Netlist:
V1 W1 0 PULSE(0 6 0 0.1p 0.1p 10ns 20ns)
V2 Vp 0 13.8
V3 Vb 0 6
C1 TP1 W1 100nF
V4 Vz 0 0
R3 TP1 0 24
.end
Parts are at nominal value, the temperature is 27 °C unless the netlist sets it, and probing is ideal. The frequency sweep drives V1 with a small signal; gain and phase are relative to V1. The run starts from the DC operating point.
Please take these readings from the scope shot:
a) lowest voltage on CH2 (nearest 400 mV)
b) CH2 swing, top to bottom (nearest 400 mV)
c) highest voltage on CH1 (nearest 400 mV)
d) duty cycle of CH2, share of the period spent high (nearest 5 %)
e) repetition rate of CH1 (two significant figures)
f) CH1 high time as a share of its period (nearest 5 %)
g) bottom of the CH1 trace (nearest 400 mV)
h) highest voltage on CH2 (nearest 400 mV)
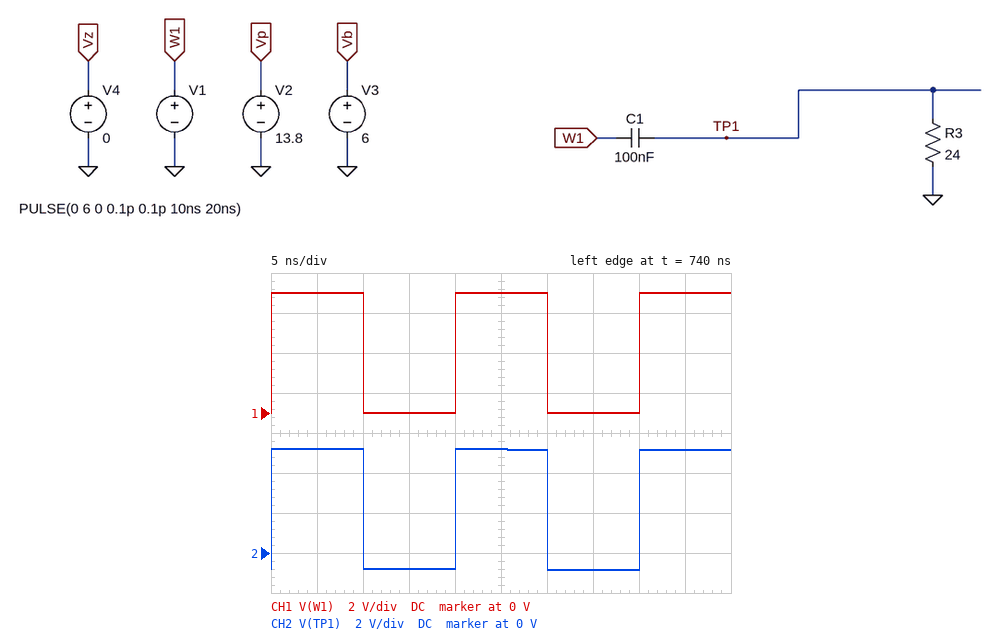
-800 mV
6.0 V
6.0 V
50 %
50 MHz
50 %
0 V
5.2 V
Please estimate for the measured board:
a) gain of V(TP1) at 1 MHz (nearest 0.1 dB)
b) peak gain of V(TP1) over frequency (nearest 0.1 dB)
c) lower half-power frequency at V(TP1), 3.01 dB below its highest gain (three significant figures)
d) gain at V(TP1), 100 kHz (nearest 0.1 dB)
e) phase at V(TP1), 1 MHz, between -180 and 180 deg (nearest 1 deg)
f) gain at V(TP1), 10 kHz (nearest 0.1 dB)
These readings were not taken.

0 dB
0 dB
66.3 kHz
-1.6 dB
4 deg
-16.5 dB
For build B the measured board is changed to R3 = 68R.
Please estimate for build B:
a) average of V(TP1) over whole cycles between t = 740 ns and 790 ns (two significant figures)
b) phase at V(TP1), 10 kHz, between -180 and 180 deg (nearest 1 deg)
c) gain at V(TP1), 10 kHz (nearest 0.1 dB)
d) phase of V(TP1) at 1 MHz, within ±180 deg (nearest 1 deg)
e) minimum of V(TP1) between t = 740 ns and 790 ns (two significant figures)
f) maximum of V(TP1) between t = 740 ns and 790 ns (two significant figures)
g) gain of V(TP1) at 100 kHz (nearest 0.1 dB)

2.7 V
67 deg
-8.1 dB
1 deg
-330 mV
5.7 V
-0.2 dB
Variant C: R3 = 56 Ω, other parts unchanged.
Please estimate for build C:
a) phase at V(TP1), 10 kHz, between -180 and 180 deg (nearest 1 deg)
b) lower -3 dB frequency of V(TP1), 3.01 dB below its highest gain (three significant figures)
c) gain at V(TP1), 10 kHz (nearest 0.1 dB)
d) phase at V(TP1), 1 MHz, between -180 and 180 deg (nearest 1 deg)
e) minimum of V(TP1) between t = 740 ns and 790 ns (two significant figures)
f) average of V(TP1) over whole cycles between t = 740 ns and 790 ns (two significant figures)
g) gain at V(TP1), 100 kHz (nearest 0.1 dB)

71 deg
28.4 kHz
-9.6 dB
2 deg
-400 mV
2.6 V
-0.3 dB
